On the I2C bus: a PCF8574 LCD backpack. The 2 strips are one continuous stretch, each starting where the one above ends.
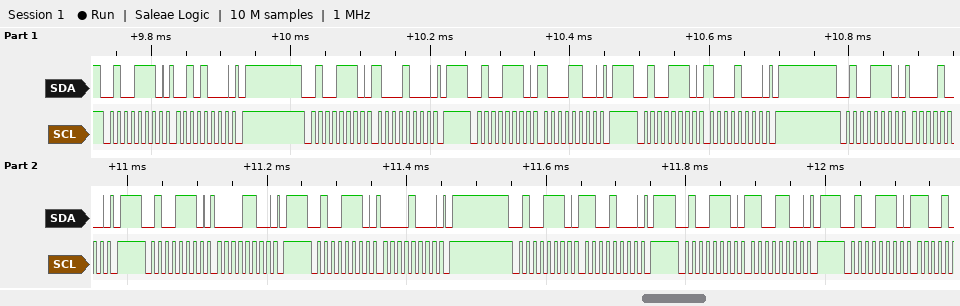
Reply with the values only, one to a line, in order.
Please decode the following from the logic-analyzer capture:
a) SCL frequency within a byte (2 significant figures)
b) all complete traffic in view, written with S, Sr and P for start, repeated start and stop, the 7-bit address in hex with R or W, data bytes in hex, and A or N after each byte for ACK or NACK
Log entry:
100 kHz
S 27W A 28 A P S 27W A 88 A P S 27W A 8C A P S 27W A 88 A P S 27W A 08 A P S 27W A 0C A P S 27W A 08 A P S 27W A C8 A P S 27W A CC A P S 27W A
